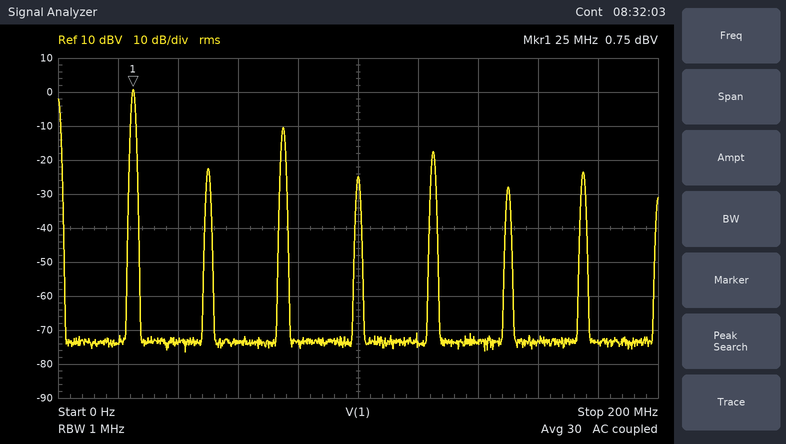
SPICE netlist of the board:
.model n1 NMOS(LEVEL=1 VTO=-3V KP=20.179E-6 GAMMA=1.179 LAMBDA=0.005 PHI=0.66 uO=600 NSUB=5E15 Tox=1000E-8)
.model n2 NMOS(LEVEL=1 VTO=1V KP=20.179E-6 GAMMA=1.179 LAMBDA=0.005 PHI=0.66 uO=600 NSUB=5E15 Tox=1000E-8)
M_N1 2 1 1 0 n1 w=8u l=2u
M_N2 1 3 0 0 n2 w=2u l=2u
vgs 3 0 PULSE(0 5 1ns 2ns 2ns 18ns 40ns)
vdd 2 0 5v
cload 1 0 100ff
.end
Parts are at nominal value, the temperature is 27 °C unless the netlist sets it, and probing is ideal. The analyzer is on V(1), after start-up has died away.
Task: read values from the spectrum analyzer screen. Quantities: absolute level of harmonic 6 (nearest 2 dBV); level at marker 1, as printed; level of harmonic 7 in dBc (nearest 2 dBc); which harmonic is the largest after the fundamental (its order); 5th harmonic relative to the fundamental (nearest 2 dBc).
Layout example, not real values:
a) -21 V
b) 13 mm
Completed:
a) -28 dBV
b) 0.75 dBV
c) -24 dBc
d) 3
e) -18 dBc
